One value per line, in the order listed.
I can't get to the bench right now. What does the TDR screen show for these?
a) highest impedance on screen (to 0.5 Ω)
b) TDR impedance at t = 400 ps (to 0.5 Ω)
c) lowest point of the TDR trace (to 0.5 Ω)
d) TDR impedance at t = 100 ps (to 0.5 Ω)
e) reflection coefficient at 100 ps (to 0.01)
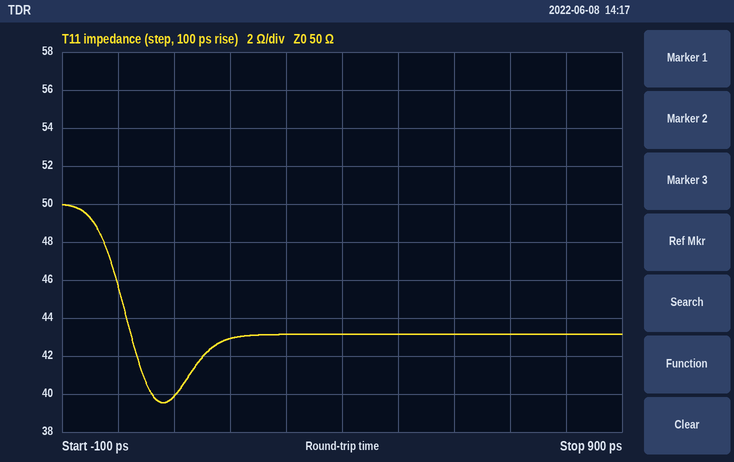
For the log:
50.0 Ω
43.0 Ω
39.5 Ω
40.0 Ω
-0.11
